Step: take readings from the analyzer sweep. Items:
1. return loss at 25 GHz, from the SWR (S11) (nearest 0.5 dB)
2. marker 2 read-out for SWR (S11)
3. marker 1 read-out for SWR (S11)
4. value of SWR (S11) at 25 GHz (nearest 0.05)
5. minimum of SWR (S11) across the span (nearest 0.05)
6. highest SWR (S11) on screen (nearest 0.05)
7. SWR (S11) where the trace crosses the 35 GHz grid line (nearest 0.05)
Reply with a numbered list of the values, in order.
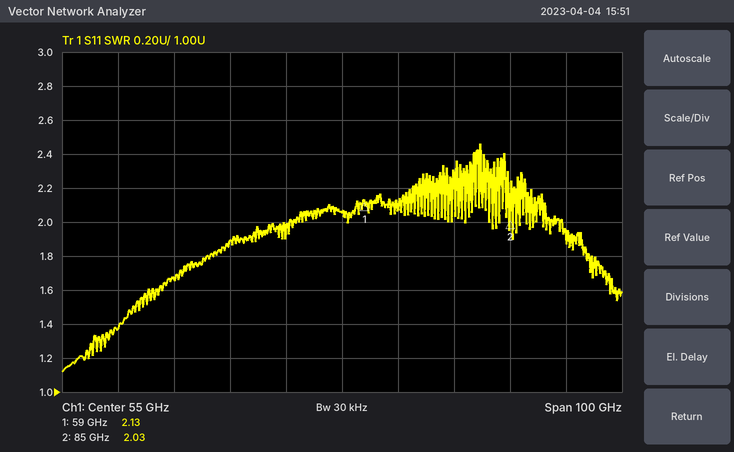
1. 12.0 dB
2. 2.03
3. 2.13
4. 1.65
5. 1.10
6. 2.45
7. 1.90
